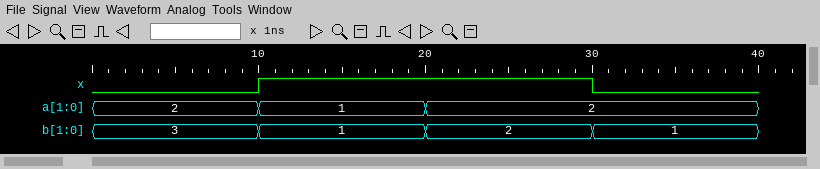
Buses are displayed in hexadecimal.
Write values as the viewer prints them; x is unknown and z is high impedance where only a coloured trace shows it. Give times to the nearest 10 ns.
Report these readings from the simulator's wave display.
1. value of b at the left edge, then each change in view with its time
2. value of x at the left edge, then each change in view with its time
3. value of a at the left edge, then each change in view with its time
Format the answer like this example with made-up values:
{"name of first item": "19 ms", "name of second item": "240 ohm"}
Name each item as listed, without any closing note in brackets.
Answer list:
{"value of b at the left edge, then each change in view with its time": "3, 1 at 10 ns, 2 at 20 ns, 1 at 30 ns", "value of x at the left edge, then each change in view with its time": "0, 1 at 10 ns, 0 at 30 ns", "value of a at the left edge, then each change in view with its time": "2, 1 at 10 ns, 2 at 20 ns"}
